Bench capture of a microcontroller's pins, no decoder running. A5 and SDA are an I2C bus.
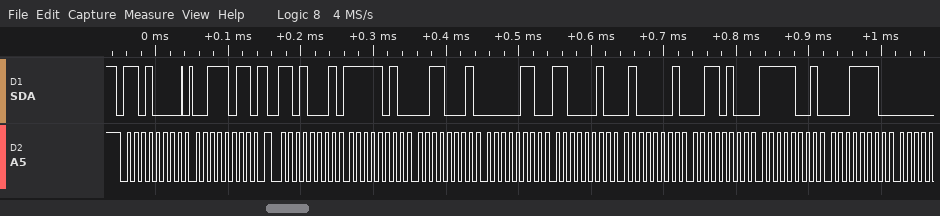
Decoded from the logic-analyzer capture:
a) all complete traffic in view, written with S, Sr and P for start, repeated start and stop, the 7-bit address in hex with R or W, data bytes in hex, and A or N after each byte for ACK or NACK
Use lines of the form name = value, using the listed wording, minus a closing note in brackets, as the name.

all complete traffic in view, written with S, Sr and P for start, repeated start and stop, the 7-bit address in hex with R or W, data bytes in hex, and A or N after each byte for ACK or NACK = S 68W A 3B A Sr 68R A FA A 31 A 06 A C2 A 41 A 34 A F9 A 1E A
